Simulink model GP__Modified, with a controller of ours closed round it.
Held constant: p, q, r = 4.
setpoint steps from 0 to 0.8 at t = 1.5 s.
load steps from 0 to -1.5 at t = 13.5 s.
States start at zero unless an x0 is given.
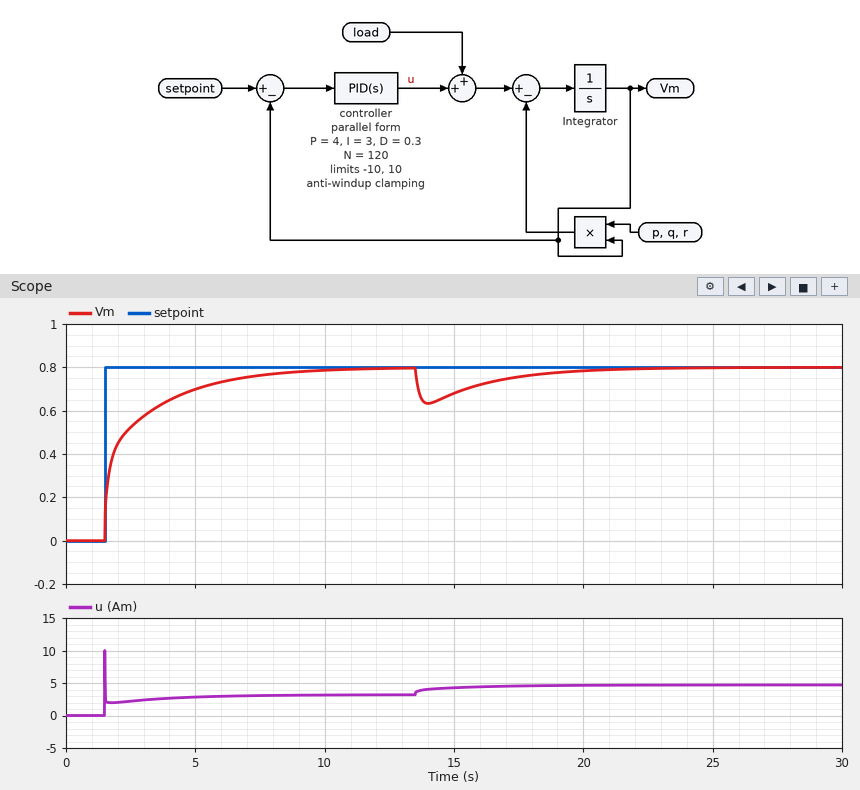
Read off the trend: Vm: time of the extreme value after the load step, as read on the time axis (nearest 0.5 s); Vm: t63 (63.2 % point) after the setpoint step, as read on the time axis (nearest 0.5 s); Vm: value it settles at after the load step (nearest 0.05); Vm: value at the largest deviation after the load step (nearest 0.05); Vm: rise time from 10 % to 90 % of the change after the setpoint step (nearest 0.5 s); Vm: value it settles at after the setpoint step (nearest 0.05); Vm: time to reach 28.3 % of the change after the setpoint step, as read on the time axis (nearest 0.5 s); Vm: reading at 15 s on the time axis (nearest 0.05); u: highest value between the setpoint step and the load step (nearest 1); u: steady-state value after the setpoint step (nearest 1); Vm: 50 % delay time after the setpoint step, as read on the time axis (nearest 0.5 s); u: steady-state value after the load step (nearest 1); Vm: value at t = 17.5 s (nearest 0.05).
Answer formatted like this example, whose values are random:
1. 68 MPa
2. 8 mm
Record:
1. 14.0 s
2. 2.5 s
3. 0.80
4. 0.65
5. 4.0 s
6. 0.80
7. 1.5 s
8. 0.70
9. 10
10. 3
11. 2.0 s
12. 5
13. 0.75
